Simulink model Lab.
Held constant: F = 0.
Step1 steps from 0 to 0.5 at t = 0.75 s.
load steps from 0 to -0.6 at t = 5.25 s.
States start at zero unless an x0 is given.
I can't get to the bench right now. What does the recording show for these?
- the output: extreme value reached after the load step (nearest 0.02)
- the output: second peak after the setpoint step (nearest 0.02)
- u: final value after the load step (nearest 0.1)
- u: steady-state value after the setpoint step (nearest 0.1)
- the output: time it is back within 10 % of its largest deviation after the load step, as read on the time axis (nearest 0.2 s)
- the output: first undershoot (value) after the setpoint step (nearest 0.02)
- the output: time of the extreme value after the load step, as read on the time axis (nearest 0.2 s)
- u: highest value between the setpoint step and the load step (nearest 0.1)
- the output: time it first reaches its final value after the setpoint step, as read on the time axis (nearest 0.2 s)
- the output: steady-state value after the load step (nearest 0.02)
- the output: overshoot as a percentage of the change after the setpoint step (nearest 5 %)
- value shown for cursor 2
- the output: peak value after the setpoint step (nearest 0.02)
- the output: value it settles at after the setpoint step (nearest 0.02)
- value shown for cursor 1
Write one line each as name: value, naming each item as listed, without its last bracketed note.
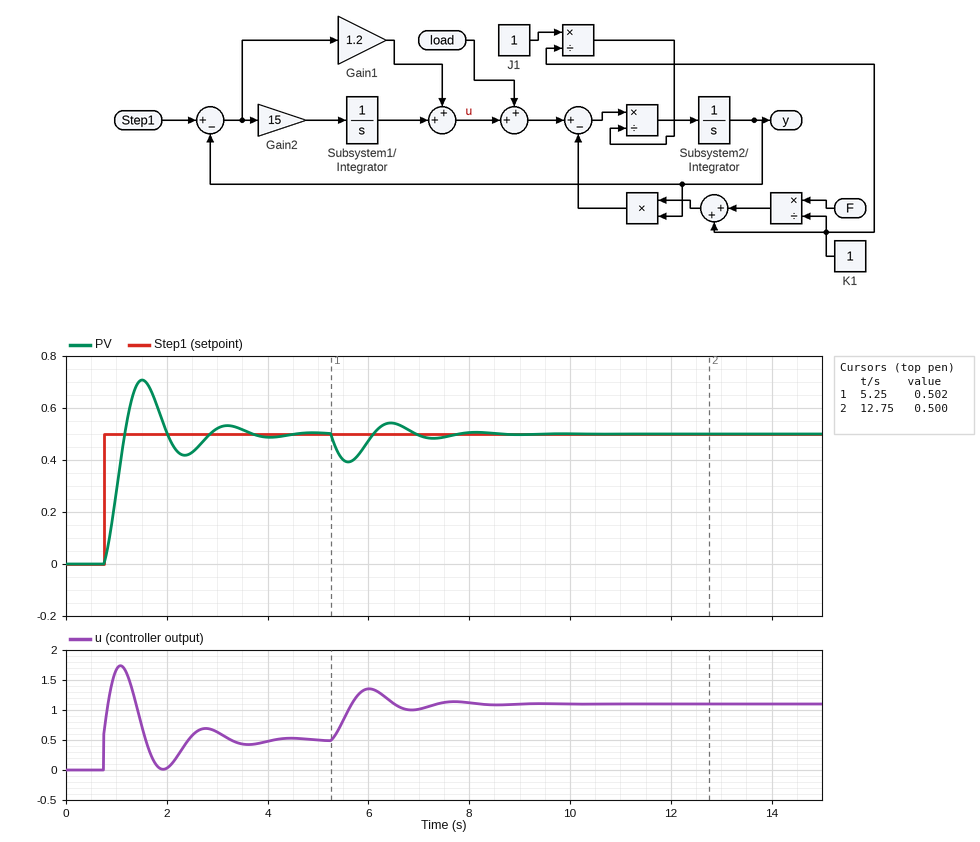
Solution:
the output: extreme value reached after the load step: 0.40
the output: second peak after the setpoint step: 0.54
u: final value after the load step: 1.1
u: steady-state value after the setpoint step: 0.5
the output: time it is back within 10 % of its largest deviation after the load step, as read on the time axis: 7.6 s
the output: first undershoot (value) after the setpoint step: 0.42
the output: time of the extreme value after the load step, as read on the time axis: 5.6 s
u: highest value between the setpoint step and the load step: 1.7
the output: time it first reaches its final value after the setpoint step, as read on the time axis: 1.2 s
the output: steady-state value after the load step: 0.50
the output: overshoot as a percentage of the change after the setpoint step: 40 %
value shown for cursor 2: 0.500
the output: peak value after the setpoint step: 0.70
the output: value it settles at after the setpoint step: 0.50
value shown for cursor 1: 0.502
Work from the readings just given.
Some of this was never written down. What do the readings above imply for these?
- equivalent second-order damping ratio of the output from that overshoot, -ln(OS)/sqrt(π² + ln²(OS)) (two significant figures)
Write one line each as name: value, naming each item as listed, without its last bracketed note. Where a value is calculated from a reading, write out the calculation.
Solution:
equivalent second-order damping ratio of the output from that overshoot, -ln(OS)/sqrt(π² + ln²(OS)): ln(0.4) = -0.916; 0.916 / sqrt(9.870 + 0.840) = 0.28
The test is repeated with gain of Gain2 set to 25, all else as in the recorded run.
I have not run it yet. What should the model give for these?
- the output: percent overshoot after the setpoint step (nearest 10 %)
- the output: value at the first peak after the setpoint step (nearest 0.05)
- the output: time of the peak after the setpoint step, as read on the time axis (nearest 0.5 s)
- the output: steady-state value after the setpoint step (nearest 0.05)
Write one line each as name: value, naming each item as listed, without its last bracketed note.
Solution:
the output: percent overshoot after the setpoint step: 50 %
the output: value at the first peak after the setpoint step: 0.75
the output: time of the peak after the setpoint step, as read on the time axis: 1.5 s
the output: steady-state value after the setpoint step: 0.50
